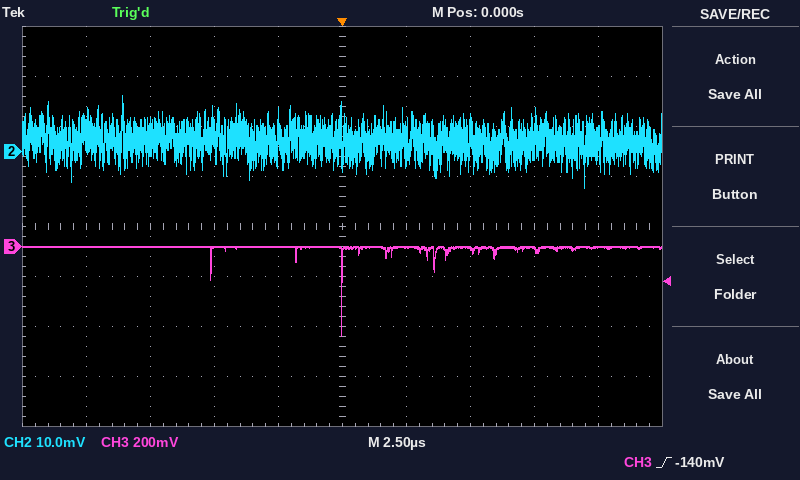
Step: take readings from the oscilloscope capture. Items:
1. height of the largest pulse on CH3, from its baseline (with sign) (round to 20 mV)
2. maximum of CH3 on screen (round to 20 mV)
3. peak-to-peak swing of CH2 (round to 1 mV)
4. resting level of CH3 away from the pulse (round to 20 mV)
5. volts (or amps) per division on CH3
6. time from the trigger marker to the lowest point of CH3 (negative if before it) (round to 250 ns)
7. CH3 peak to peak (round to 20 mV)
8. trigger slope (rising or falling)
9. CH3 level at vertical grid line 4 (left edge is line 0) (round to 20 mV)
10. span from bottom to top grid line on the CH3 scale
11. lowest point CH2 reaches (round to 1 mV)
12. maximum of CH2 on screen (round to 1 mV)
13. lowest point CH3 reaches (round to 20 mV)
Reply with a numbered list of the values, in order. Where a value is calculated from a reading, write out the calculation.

1. -360 mV − (0 mV) = -360 mV
2. 0 mV
3. 11 mV − (-7 mV) = 18 mV
4. 0 mV
5. 200 mV
6. 0.00 µs
7. 0 mV − (-360 mV) = 360 mV
8. rising
9. 0 mV
10. 1.6 V
11. -7 mV
12. 11 mV
13. -360 mV
